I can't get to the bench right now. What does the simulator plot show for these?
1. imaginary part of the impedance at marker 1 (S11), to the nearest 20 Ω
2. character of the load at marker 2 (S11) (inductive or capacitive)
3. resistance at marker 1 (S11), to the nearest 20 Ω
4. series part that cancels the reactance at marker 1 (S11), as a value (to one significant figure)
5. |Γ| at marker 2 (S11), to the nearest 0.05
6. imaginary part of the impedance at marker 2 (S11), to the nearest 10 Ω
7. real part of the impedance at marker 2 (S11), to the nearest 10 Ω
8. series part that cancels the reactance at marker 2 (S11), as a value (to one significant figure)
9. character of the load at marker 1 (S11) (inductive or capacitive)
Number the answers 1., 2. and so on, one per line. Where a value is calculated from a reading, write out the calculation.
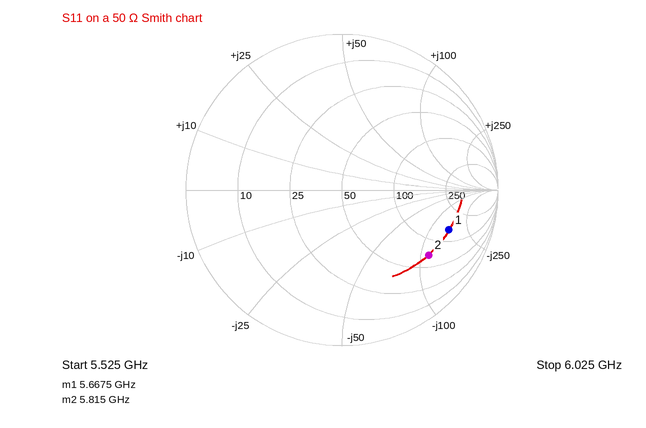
1. -160 Ω
2. capacitive
3. 140 Ω
4. L = 160 Ω/(2π × 5.6675 GHz) ≈ 4 nH
5. 0.70
6. -110 Ω
7. 70 Ω
8. L = 110 Ω/(2π × 5.815 GHz) ≈ 3 nH
9. capacitive
